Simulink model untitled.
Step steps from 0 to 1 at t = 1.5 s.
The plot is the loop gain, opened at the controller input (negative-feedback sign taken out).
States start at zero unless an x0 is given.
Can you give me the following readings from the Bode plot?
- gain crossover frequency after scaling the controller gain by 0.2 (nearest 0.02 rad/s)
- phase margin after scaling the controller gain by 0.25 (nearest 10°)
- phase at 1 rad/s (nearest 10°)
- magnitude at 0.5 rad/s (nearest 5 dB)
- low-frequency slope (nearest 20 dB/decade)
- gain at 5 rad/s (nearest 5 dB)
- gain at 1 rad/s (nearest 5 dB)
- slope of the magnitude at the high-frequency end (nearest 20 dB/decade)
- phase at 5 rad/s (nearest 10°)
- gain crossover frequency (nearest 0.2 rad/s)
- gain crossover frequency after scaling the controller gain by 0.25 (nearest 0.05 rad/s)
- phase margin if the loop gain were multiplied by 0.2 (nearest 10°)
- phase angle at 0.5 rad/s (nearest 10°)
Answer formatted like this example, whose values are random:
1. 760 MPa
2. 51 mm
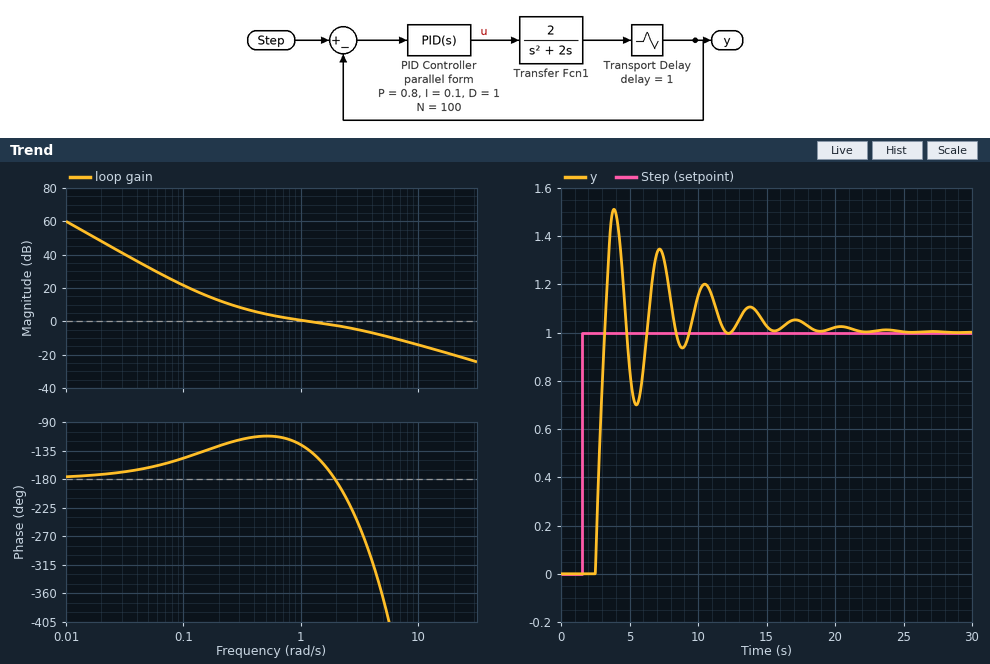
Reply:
1. 0.18 rad/s
2. 50°
3. -130°
4. 5 dB
5. -40 dB/decade
6. -10 dB
7. 0 dB
8. -20 dB/decade
9. -370°
10. 1.2 rad/s
11. 0.20 rad/s
12. 50°
13. -110°
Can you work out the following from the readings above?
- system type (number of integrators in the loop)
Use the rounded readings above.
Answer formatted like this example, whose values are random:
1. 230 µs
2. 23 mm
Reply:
1. 2
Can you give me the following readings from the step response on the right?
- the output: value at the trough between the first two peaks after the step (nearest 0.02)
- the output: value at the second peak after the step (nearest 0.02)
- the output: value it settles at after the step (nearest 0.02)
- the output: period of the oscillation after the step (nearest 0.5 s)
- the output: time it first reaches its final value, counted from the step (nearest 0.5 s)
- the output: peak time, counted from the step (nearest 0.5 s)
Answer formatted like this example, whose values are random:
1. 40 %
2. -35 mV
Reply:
1. 0.70
2. 1.34
3. 1.00
4. 3.5 s
5. 1.5 s
6. 2.5 s
